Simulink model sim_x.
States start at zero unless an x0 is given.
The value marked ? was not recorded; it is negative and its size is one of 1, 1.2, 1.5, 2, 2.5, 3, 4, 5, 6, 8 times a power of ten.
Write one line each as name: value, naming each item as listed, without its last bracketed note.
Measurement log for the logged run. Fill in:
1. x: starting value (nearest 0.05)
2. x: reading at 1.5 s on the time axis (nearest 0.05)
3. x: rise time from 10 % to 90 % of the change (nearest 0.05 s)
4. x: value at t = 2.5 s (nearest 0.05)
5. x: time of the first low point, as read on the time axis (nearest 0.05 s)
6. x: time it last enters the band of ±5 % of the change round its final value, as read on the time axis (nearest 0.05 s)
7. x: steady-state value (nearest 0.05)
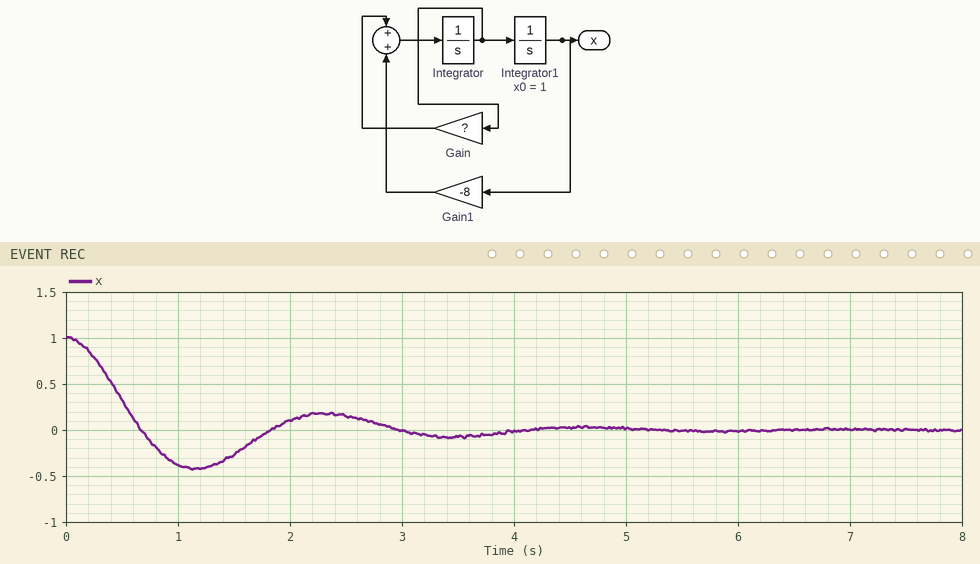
x: starting value: 1.00
x: reading at 1.5 s on the time axis: -0.25
x: rise time from 10 % to 90 % of the change: 0.45 s
x: value at t = 2.5 s: 0.15
x: time of the first low point, as read on the time axis: 1.15 s
x: time it last enters the band of ±5 % of the change round its final value, as read on the time axis: 3.80 s
x: steady-state value: 0.00
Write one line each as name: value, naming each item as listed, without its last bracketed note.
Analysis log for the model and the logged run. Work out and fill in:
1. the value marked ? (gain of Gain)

the value marked ?: -1.5
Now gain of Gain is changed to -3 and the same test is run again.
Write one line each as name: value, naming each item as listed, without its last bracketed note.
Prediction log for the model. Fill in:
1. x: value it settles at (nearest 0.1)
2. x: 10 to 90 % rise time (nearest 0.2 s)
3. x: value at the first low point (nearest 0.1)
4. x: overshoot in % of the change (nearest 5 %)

x: value it settles at: 0.0
x: 10 to 90 % rise time: 0.6 s
x: value at the first low point: -0.1
x: overshoot in % of the change: 15 %
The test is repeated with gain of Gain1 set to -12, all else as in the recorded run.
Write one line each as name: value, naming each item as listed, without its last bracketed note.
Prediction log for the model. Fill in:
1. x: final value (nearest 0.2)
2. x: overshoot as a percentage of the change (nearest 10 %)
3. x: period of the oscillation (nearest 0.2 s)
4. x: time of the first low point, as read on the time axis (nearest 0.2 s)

x: final value: 0.0
x: overshoot as a percentage of the change: 50 %
x: period of the oscillation: 1.8 s
x: time of the first low point, as read on the time axis: 1.0 s
